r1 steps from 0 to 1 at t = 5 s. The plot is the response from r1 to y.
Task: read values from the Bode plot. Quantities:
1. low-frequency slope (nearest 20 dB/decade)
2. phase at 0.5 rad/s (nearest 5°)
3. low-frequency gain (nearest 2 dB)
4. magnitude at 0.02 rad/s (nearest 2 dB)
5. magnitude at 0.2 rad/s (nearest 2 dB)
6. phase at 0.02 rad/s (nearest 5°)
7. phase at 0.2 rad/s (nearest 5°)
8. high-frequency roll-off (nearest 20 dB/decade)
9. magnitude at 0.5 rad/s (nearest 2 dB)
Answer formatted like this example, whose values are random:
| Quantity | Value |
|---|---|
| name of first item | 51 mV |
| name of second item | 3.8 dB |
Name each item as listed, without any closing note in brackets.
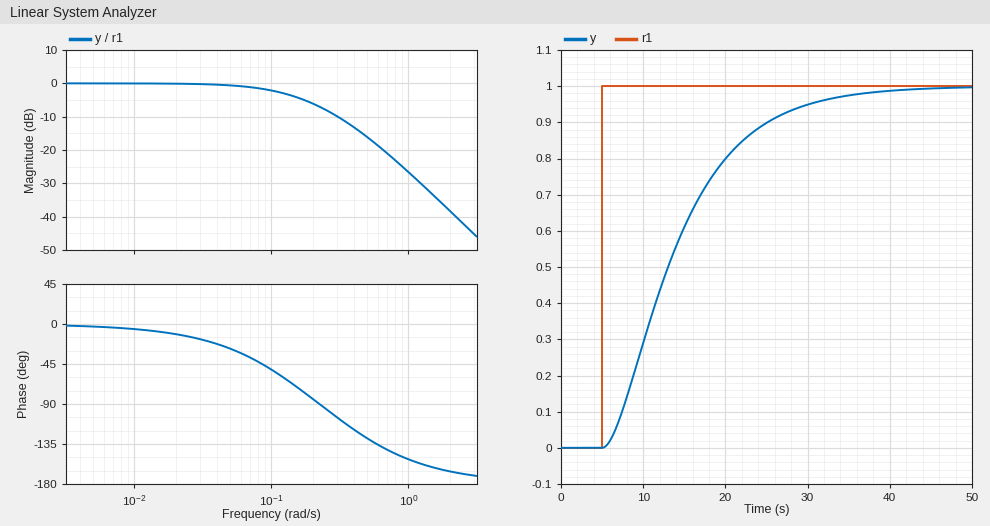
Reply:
| Quantity | Value |
|---|---|
| low-frequency slope | 0 dB/decade |
| phase at 0.5 rad/s | -130° |
| low-frequency gain | 0 dB |
| magnitude at 0.02 rad/s | 0 dB |
| magnitude at 0.2 rad/s | -6 dB |
| phase at 0.02 rad/s | -10° |
| phase at 0.2 rad/s | -85° |
| high-frequency roll-off | -40 dB/decade |
| magnitude at 0.5 rad/s | -16 dB |
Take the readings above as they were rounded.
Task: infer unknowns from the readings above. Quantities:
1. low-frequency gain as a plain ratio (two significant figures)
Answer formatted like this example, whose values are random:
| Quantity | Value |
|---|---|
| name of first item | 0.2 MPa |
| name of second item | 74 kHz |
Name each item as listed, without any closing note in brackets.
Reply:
| Quantity | Value |
|---|---|
| low-frequency gain as a plain ratio | 1.0 |
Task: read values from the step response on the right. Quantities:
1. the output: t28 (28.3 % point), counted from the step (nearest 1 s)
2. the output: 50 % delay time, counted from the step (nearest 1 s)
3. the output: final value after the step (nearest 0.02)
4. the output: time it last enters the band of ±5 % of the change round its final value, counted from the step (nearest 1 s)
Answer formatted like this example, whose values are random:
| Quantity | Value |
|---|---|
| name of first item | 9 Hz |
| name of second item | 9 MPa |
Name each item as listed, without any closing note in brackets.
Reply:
| Quantity | Value |
|---|---|
| the output: t28 (28.3 % point), counted from the step | 5 s |
| the output: 50 % delay time, counted from the step | 8 s |
| the output: final value after the step | 1.00 |
| the output: time it last enters the band of ±5 % of the change round its final value, counted from the step | 25 s |
